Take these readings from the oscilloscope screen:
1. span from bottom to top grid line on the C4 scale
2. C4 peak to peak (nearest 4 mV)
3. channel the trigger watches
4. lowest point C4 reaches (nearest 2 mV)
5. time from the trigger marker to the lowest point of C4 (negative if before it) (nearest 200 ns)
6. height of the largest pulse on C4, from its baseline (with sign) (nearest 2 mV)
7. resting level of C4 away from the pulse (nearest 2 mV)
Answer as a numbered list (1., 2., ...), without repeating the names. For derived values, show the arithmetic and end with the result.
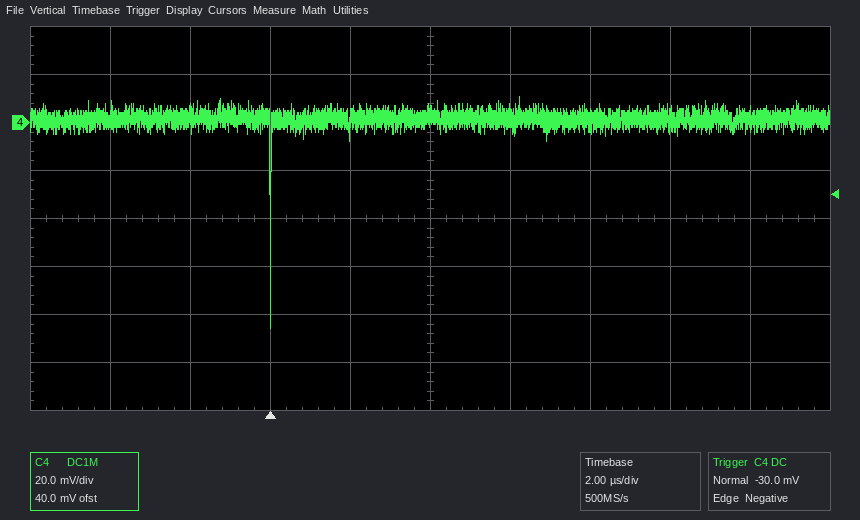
1. 160 mV
2. 96 mV
3. C4
4. -86 mV
5. 0.0 µs
6. -86 mV − (2 mV) = -88 mV
7. 2 mV
